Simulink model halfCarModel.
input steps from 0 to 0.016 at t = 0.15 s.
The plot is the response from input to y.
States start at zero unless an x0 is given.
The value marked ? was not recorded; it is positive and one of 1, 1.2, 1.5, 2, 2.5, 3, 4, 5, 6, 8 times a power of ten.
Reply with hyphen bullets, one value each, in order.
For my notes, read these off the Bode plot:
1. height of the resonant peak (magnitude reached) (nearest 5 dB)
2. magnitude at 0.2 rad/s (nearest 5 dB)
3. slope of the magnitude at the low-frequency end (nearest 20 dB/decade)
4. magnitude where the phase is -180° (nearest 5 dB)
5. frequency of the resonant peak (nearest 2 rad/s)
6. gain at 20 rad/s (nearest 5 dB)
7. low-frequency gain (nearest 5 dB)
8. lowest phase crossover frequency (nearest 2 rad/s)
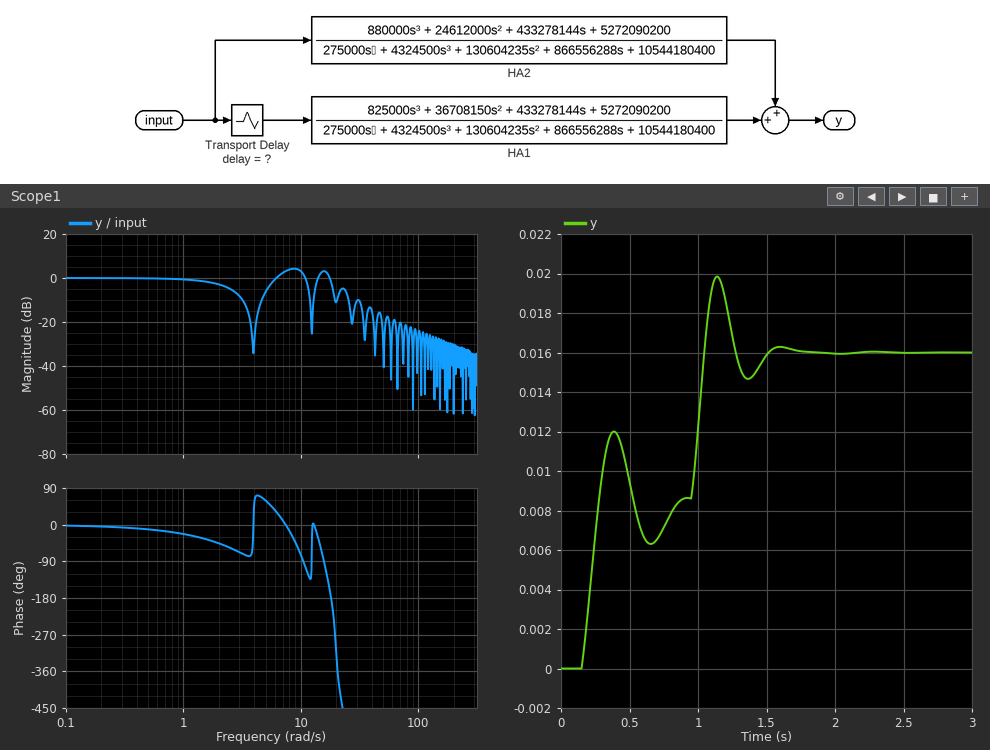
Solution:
- 5 dB
- 0 dB
- 0 dB/decade
- 0 dB
- 8 rad/s
- -10 dB
- 0 dB
- 18 rad/s
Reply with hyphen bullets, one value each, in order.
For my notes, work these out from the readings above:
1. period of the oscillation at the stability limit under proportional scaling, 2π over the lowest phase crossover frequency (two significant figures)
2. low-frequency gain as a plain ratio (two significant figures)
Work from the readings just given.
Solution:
- 0.35 s
- 1.0
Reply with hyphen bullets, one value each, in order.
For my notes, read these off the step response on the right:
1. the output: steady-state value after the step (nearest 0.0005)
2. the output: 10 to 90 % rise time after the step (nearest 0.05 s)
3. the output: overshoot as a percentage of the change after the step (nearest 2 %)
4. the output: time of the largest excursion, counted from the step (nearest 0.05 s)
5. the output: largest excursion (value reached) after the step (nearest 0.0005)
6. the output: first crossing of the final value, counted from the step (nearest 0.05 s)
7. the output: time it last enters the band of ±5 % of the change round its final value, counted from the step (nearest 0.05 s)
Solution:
- 0.0160
- 0.85 s
- 24 %
- 1.00 s
- 0.0200
- 0.90 s
- 1.30 s
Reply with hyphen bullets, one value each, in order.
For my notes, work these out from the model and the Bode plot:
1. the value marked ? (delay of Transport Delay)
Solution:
- 0.8
